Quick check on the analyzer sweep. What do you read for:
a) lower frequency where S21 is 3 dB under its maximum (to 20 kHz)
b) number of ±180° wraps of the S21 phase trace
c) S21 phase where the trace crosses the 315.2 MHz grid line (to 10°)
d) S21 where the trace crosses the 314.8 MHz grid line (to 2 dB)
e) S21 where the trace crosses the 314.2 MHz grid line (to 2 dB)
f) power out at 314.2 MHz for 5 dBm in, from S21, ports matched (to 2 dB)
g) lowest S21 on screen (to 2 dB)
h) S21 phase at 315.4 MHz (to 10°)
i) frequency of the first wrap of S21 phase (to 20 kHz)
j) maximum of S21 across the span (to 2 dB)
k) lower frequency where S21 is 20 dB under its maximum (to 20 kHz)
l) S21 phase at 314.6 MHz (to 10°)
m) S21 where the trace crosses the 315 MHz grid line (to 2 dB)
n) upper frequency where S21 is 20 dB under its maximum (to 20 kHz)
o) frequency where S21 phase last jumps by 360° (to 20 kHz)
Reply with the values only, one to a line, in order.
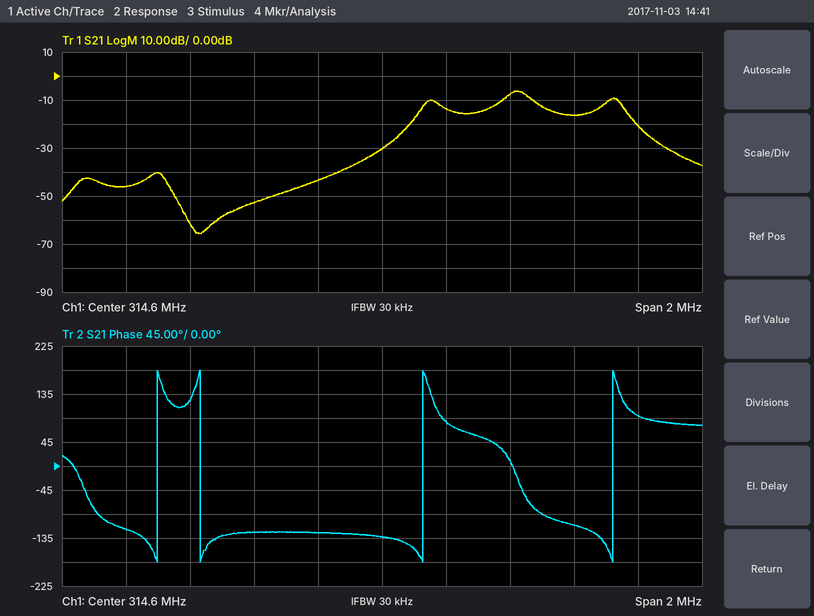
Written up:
314.98 MHz
4
-110°
-14 dB
-52 dB
-48 dBm
-66 dB
90°
313.90 MHz
-6 dB
314.64 MHz
-130°
-8 dB
315.44 MHz
315.32 MHz
